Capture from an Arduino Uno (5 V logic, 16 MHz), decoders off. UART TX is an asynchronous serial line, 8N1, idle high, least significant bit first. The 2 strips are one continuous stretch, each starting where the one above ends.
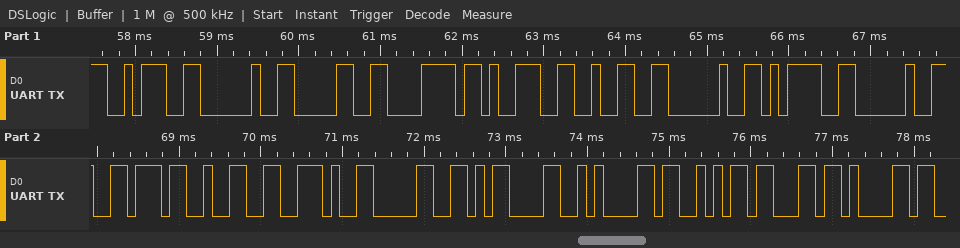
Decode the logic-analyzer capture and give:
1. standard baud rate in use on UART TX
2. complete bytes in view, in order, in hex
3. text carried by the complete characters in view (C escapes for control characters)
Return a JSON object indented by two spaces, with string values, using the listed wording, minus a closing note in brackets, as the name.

{
  "standard baud rate in use on UART TX": "9600 baud",
  "complete bytes in view, in order, in hex": "3A 20 30 78 39 32 20 3D 20 76 32 2E 30 0D 0A 53 63 61",
  "text carried by the complete characters in view": "\": 0x92 = v2.0\\r\\nSca\""
}
